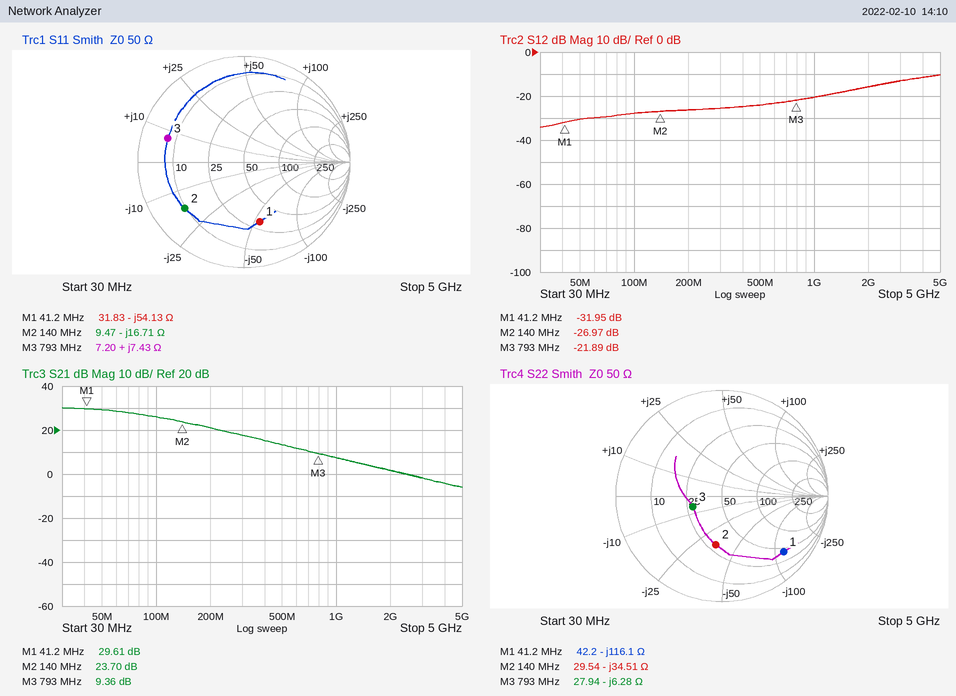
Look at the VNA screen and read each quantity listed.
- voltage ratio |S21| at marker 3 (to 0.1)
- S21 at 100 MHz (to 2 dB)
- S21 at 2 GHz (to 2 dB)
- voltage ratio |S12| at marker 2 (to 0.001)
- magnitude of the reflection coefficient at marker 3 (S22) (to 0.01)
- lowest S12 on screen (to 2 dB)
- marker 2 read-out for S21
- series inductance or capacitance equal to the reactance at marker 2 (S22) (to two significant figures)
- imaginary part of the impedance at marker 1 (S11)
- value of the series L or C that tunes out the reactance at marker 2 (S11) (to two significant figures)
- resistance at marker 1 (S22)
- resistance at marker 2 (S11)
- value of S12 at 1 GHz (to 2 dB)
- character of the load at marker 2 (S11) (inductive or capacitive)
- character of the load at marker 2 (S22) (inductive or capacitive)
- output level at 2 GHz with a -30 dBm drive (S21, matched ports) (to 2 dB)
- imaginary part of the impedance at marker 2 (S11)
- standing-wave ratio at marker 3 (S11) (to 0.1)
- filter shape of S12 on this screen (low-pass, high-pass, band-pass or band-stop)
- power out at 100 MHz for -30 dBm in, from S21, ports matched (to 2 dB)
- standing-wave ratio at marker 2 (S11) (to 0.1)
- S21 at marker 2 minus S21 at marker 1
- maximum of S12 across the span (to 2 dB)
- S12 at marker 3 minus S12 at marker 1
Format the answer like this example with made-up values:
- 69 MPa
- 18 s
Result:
- 2.9
- 26 dB
- 2 dB
- 0.045
- 0.29
- -34 dB
- 23.70 dB
- 33 pF
- -54.13 Ω
- 19 nH
- 42.2 Ω
- 9.47 Ω
- -20 dB
- capacitive
- capacitive
- -28 dBm
- -16.71 Ω
- 7.1
- high-pass
- -4 dBm
- 5.9
- -5.91 dB
- -10 dB
- 10.06 dB
